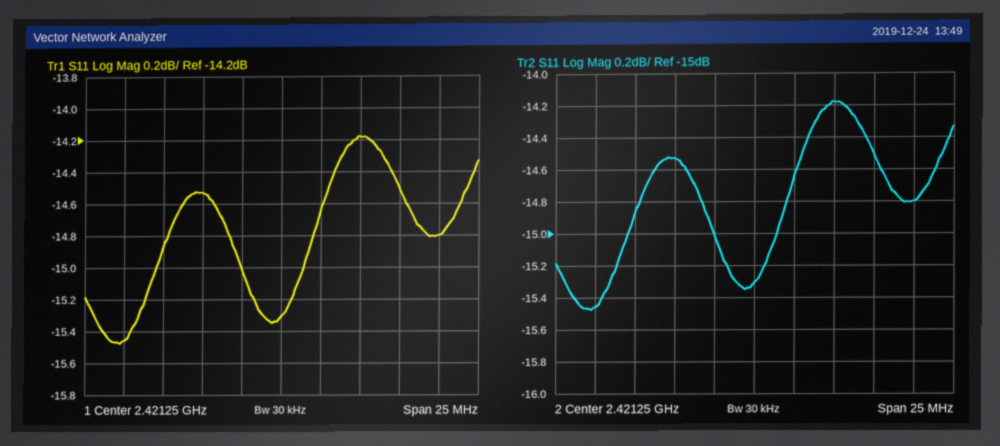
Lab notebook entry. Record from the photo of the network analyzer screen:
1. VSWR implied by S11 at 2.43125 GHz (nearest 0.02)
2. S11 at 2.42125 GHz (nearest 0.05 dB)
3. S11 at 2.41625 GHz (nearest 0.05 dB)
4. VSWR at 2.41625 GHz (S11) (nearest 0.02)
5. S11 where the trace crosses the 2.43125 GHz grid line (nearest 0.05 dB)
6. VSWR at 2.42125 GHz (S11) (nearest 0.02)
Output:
1.44
-15.30 dB
-14.55 dB
1.46
-14.80 dB
1.42
